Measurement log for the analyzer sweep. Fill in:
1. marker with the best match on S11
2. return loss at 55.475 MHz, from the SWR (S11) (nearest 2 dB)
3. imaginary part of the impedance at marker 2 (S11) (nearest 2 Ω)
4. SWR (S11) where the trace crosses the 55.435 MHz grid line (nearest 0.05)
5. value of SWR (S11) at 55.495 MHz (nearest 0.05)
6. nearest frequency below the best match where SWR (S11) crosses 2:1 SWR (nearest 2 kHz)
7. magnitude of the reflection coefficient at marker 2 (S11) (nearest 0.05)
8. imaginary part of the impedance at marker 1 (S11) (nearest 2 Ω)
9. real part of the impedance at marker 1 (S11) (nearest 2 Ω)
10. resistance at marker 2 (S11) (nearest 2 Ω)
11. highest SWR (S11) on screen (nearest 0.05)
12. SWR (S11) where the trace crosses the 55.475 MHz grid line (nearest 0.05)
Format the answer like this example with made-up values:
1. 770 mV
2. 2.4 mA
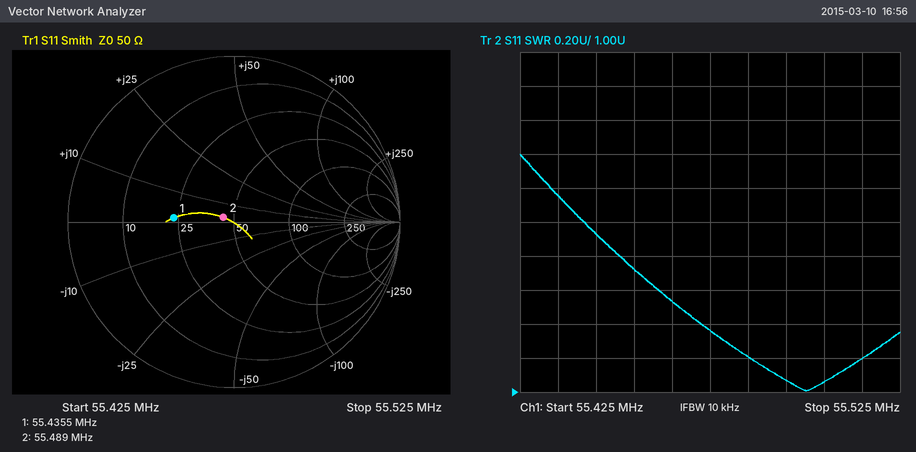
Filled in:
1. marker 2
2. 16 dB
3. +2 Ω
4. 2.15
5. 1.05
6. 55.442 MHz
7. 0.05
8. +2 Ω
9. 24 Ω
10. 44 Ω
11. 2.40
12. 1.35
